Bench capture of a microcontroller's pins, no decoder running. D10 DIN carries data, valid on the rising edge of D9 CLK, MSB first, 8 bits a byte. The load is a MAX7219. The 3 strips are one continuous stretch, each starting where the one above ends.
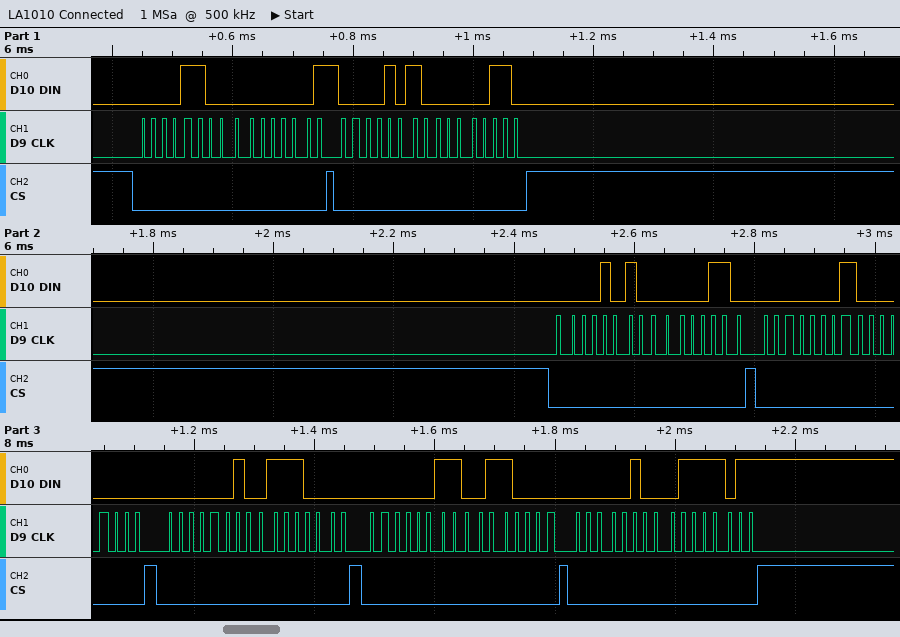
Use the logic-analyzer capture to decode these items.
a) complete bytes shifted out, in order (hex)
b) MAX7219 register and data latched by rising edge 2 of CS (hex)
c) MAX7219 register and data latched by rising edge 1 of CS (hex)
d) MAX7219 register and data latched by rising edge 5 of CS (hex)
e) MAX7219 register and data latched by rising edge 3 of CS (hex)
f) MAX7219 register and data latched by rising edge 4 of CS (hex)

0x0C 0x01 0x0A 0x06 0x0A 0x06 0x01 0x00 0x02 0x70 0x03 0x30 0x04 0x7B
register 0xA, data 0x06
register 0xC, data 0x01
register 0x2, data 0x70
register 0xA, data 0x06
register 0x1, data 0x00
